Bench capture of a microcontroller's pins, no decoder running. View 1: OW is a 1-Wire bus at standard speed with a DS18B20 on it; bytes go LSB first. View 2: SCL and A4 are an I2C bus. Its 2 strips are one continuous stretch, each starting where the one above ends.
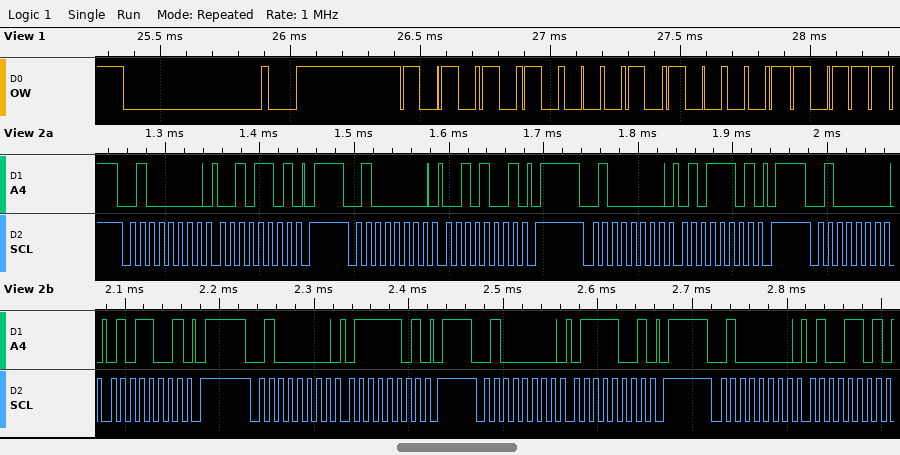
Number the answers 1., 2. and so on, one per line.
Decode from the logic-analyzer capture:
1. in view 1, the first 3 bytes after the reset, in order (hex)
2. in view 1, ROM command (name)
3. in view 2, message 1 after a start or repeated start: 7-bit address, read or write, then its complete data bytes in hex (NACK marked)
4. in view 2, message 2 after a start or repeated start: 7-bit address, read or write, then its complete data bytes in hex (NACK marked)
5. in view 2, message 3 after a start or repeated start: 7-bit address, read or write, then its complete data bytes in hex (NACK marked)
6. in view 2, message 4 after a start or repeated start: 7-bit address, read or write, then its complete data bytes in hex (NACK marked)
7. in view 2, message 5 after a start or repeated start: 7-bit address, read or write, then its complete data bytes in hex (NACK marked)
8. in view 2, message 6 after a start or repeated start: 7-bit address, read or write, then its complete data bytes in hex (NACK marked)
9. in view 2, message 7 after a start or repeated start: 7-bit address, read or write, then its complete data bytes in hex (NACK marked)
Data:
1. 55 28 EC
2. Match ROM
3. 0x20 write: 2D
4. 0x20 write: 29
5. 0x20 write: 5D
6. 0x20 write: 59
7. 0x20 write: 7D
8. 0x20 write: 79
9. 0x20 write: 4D
